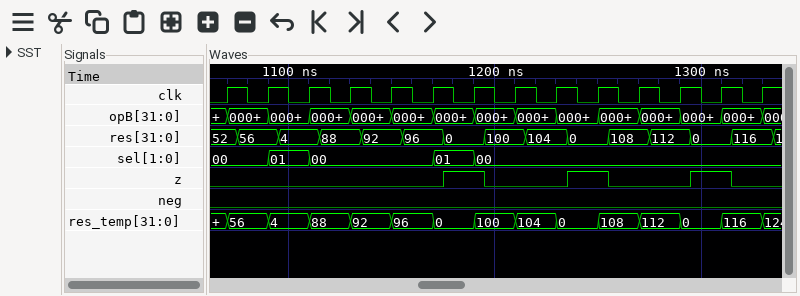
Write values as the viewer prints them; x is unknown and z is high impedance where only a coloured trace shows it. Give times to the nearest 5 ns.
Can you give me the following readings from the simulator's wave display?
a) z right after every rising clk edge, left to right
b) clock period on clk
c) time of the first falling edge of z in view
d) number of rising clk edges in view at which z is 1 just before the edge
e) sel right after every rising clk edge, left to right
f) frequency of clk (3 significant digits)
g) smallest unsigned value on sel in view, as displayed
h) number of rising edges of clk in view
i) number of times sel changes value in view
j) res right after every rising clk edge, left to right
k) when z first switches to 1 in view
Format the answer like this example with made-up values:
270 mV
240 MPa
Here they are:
0 0 0 0 0 0 1 0 0 1 0 0 1 0
20 ns
1195 ns
3
00, 01, 00, 00, 00, 01, 00, 00, 00, 00, 00, 00, 00, 00
50.0 MHz
00
14
4
52, 56, 4, 88, 92, 96, 0, 100, 104, 0, 108, 112, 0, 116
1175 ns
